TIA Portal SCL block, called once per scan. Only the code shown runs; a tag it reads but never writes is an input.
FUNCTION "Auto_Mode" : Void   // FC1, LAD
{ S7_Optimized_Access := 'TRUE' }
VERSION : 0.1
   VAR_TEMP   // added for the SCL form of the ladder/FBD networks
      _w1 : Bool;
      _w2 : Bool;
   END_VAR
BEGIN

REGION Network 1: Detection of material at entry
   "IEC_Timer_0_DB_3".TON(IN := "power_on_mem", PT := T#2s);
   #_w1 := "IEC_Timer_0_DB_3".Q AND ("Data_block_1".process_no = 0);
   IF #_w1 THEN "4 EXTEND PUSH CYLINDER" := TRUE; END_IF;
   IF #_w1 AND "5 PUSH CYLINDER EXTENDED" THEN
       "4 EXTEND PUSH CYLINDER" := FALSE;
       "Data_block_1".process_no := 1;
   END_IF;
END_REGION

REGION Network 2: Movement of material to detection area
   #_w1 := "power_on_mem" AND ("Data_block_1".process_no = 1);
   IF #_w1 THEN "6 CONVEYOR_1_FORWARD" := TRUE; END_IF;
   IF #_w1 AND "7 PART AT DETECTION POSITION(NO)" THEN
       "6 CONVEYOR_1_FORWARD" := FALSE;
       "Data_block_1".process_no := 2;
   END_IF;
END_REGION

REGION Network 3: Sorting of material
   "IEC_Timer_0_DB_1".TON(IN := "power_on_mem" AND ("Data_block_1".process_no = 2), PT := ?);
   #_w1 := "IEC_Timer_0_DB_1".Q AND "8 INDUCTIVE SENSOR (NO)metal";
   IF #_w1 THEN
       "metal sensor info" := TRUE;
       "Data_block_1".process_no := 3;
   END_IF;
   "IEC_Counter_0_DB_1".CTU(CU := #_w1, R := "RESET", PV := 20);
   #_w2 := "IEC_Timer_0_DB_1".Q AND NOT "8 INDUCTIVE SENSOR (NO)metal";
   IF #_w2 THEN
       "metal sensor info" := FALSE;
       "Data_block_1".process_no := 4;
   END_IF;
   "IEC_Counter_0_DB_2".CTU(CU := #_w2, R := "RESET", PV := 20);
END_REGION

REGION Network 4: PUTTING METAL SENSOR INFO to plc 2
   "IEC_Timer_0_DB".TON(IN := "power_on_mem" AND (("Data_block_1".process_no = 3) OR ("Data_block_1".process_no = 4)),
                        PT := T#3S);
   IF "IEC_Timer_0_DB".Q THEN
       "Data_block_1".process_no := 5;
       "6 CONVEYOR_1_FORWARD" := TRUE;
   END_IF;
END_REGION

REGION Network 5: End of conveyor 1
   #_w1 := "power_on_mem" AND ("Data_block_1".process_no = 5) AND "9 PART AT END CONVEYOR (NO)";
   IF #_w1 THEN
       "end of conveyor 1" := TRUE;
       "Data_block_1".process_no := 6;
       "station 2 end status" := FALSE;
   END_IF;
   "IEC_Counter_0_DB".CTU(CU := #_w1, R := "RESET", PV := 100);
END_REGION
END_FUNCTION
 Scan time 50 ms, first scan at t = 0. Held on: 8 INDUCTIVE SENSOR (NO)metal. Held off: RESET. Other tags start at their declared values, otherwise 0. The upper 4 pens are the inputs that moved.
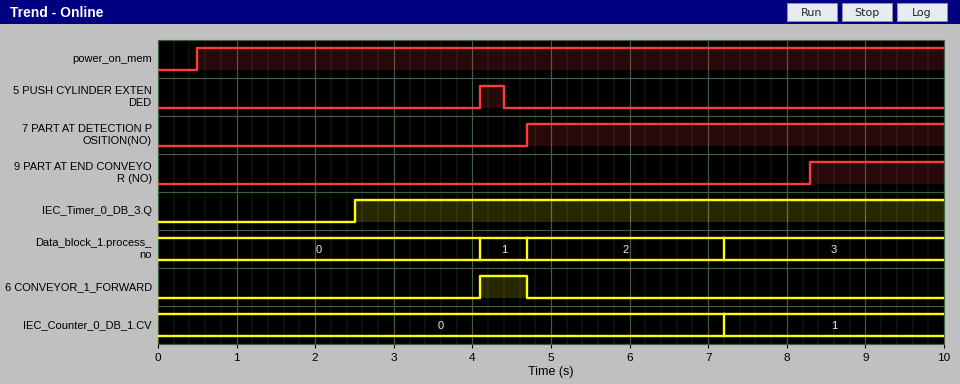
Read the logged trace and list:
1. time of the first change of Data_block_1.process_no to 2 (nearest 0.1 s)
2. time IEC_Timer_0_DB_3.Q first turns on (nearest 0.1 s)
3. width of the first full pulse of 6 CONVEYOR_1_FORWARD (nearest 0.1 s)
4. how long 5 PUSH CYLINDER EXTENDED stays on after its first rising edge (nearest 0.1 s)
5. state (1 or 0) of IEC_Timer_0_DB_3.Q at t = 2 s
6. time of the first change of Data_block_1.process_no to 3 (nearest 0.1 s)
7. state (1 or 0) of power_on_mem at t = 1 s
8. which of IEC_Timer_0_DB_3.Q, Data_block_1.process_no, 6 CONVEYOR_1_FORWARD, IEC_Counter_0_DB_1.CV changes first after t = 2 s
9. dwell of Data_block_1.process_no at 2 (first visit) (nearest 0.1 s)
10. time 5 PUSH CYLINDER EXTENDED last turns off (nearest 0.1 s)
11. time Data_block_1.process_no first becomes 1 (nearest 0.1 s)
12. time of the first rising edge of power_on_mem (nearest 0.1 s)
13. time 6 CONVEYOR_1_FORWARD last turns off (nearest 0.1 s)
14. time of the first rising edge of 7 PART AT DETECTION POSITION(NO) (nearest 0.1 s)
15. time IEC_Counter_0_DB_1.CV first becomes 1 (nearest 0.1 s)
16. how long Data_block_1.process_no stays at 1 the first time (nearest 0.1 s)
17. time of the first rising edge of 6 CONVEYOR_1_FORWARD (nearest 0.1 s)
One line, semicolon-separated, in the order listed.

4.7 s; 2.5 s; 0.6 s; 0.3 s; 0; 7.2 s; 1; IEC_Timer_0_DB_3.Q; 2.5 s; 4.4 s; 4.1 s; 0.5 s; 4.7 s; 4.7 s; 7.2 s; 0.6 s; 4.1 s
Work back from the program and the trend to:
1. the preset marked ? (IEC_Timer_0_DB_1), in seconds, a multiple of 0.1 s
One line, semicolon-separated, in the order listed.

2.5 s
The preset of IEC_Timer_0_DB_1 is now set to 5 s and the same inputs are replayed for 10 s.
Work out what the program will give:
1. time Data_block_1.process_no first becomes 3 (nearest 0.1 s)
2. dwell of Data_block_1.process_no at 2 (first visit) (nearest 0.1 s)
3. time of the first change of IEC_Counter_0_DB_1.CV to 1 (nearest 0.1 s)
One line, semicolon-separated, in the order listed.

9.7 s; 5.0 s; 9.7 s
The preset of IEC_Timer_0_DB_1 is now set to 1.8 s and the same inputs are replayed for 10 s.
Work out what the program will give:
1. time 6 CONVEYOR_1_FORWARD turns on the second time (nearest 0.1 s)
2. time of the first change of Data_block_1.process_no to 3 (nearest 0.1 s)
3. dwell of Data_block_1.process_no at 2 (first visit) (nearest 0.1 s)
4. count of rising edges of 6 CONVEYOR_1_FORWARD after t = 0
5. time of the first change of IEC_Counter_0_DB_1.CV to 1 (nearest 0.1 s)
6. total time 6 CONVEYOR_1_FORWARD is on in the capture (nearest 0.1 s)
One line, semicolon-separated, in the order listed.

9.5 s; 6.5 s; 1.8 s; 2; 6.5 s; 1.1 s
